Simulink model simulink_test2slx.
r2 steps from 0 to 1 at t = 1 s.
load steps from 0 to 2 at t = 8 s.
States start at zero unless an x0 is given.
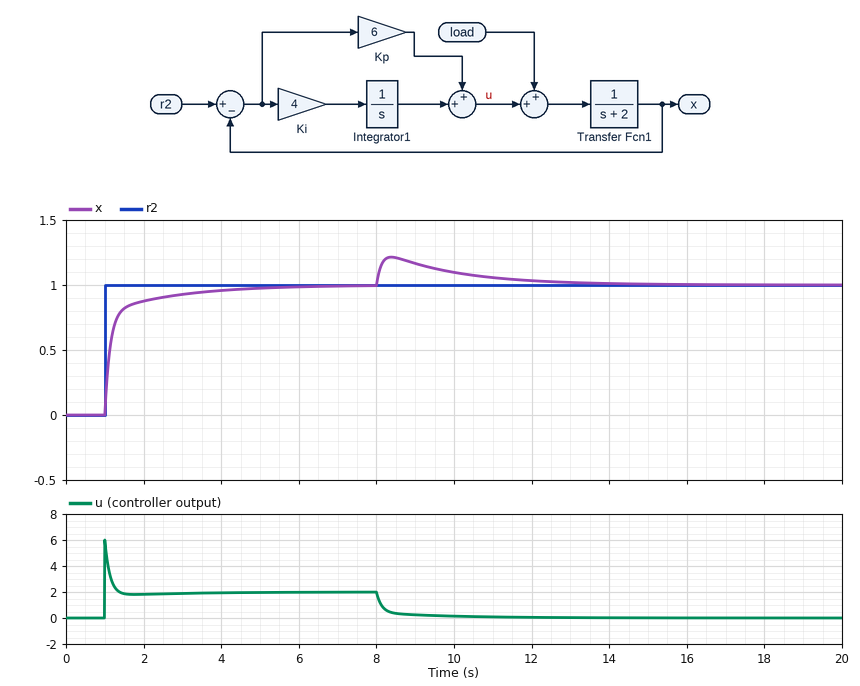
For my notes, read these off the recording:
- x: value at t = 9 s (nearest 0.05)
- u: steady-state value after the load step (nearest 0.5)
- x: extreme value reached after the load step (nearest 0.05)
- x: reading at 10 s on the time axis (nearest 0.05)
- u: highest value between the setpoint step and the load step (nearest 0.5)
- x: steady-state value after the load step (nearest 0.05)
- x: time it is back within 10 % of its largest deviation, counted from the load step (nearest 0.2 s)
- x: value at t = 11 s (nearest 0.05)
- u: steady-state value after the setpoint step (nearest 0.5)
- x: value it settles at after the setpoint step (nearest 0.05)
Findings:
1.15
0.0
1.20
1.10
6.0
1.00
4.8 s
1.05
2.0
1.00
